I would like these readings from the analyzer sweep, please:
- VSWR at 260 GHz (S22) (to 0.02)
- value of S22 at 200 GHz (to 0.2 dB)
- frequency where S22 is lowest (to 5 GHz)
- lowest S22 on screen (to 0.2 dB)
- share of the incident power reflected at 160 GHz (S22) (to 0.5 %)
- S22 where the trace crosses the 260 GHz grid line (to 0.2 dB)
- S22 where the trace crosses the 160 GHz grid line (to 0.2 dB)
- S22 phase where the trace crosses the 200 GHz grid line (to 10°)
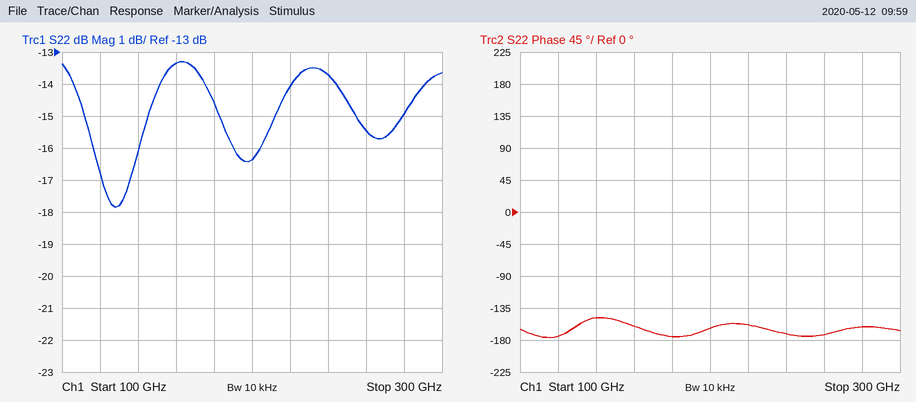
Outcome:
1.40
-16.4 dB
130 GHz
-17.8 dB
4.5 %
-15.4 dB
-13.4 dB
-160°
